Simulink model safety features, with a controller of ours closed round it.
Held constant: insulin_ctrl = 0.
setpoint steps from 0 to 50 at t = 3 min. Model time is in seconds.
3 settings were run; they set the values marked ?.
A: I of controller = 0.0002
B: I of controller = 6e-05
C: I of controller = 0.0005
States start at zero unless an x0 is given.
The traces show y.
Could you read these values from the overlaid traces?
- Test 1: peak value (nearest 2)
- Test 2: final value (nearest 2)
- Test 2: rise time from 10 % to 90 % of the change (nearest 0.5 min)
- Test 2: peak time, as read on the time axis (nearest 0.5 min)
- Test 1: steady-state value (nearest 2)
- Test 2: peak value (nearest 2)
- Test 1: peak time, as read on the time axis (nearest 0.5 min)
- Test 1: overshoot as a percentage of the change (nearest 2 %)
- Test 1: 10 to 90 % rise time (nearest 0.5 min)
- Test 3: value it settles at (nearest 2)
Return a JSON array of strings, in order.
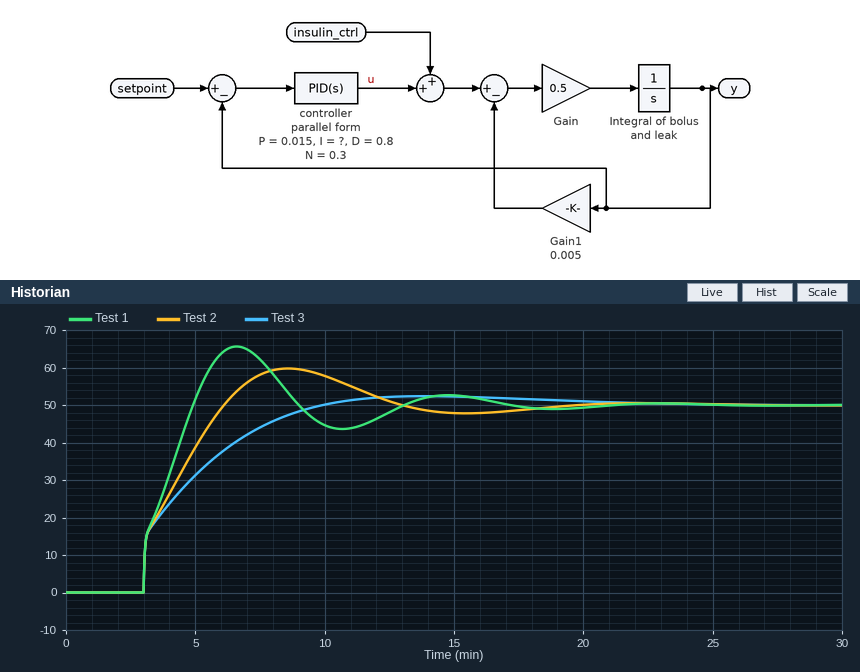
["66", "50", "2.5 min", "8.5 min", "50", "60", "6.5 min", "32 %", "1.5 min", "50"]
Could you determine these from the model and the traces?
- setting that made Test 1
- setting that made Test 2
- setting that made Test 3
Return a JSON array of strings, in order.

["C", "A", "B"]
